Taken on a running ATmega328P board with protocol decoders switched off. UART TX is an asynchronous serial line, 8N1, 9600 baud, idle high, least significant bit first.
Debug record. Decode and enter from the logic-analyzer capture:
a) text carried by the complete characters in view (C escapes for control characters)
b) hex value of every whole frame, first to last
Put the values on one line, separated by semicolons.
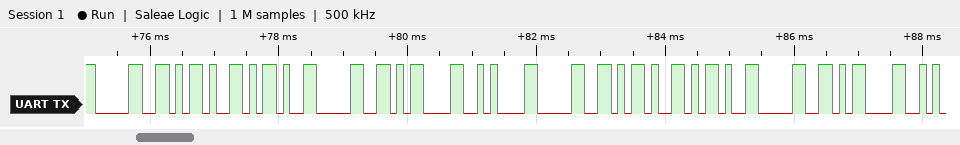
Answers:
"0--0\r\n0--0\r"; 0x30 0x2D 0x2D 0x30 0x0D 0x0A 0x30 0x2D 0x2D 0x30 0x0D
